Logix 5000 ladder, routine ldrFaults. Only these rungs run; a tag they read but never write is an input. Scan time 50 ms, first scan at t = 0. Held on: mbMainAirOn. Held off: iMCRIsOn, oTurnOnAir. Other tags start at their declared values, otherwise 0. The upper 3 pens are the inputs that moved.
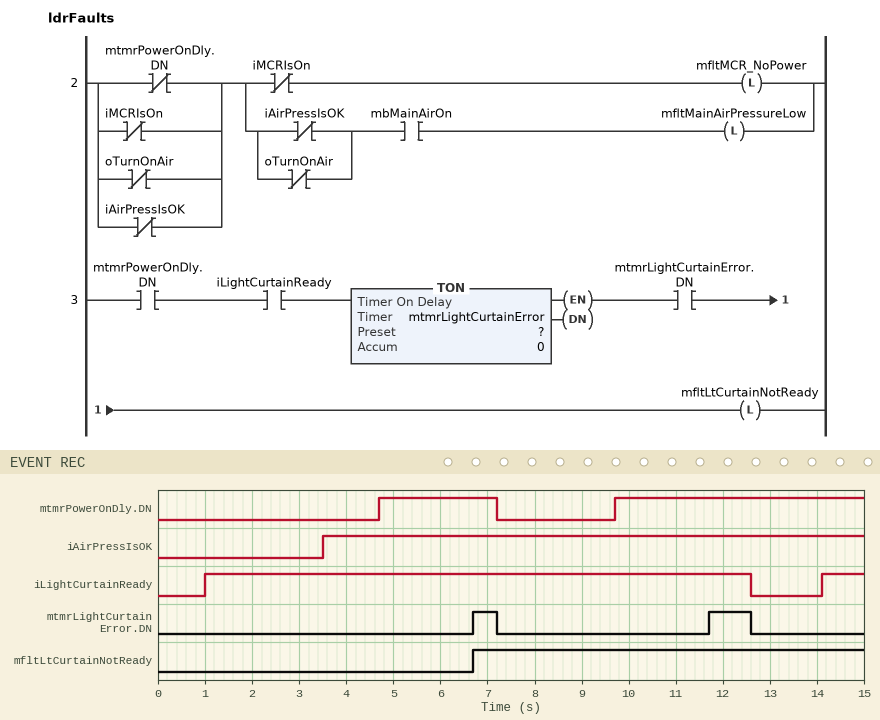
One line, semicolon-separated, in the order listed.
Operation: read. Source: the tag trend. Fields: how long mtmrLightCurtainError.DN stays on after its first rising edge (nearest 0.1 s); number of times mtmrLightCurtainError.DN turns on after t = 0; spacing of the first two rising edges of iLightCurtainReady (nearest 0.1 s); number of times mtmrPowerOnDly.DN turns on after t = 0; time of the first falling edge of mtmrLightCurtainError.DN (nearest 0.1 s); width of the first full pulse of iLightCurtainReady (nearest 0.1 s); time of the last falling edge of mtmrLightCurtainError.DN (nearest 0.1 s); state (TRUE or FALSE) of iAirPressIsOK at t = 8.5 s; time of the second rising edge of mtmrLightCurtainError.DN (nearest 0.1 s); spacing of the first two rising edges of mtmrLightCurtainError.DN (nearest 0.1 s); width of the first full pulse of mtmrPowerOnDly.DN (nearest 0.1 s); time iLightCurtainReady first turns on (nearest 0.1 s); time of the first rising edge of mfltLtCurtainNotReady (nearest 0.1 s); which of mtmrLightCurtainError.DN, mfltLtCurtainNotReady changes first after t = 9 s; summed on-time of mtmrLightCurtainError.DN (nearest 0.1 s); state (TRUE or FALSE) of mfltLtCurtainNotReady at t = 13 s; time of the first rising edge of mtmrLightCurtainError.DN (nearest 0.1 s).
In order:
0.5 s; 2; 13.1 s; 2; 7.2 s; 11.6 s; 12.6 s; TRUE; 11.7 s; 5.0 s; 2.5 s; 1.0 s; 6.7 s; mtmrLightCurtainError.DN; 1.4 s; TRUE; 6.7 s
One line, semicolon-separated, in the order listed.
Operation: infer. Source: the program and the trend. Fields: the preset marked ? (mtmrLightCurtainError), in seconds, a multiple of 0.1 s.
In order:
2.0 s
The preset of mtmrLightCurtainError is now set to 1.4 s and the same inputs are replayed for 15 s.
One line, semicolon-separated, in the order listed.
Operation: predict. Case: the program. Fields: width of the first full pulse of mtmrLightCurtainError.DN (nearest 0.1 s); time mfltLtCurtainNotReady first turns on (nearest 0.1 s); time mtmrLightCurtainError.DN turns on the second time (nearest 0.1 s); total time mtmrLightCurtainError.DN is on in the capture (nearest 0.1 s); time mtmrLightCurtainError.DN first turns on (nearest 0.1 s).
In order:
1.1 s; 6.1 s; 11.1 s; 2.6 s; 6.1 s
